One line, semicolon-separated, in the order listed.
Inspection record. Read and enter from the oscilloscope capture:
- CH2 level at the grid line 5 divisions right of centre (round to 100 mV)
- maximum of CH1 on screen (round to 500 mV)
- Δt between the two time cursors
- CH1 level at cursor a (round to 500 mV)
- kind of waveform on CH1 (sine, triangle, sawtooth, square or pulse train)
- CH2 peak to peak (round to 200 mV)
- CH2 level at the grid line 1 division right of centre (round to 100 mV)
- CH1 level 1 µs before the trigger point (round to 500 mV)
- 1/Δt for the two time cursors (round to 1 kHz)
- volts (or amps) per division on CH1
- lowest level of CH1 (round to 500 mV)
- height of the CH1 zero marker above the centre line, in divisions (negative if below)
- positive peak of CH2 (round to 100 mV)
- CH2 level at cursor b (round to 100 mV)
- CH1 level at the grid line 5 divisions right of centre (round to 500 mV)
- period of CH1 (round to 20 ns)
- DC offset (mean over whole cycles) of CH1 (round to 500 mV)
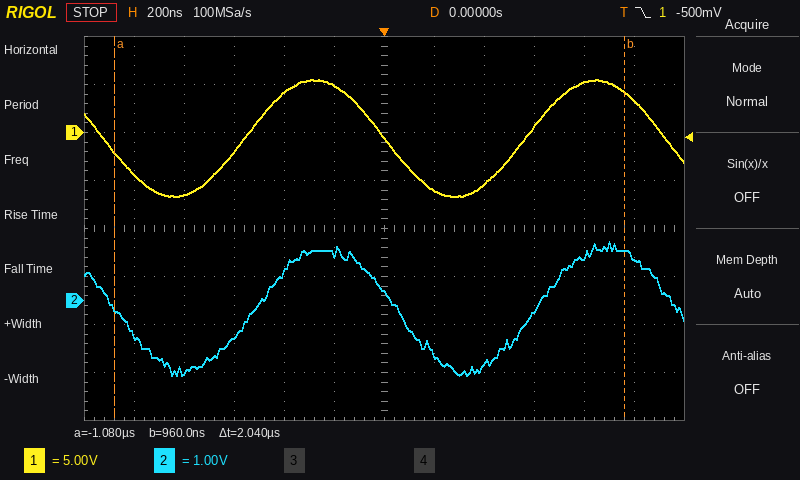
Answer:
900 mV; 5.5 V; 2.04 µs; -2.0 V; sine; 2.8 V; -1.1 V; -4.5 V; 490 kHz; 5 V; -6.5 V; +2.0 div; 1.2 V; 1.0 V; 3.5 V; 1.12 µs; -500 mV
